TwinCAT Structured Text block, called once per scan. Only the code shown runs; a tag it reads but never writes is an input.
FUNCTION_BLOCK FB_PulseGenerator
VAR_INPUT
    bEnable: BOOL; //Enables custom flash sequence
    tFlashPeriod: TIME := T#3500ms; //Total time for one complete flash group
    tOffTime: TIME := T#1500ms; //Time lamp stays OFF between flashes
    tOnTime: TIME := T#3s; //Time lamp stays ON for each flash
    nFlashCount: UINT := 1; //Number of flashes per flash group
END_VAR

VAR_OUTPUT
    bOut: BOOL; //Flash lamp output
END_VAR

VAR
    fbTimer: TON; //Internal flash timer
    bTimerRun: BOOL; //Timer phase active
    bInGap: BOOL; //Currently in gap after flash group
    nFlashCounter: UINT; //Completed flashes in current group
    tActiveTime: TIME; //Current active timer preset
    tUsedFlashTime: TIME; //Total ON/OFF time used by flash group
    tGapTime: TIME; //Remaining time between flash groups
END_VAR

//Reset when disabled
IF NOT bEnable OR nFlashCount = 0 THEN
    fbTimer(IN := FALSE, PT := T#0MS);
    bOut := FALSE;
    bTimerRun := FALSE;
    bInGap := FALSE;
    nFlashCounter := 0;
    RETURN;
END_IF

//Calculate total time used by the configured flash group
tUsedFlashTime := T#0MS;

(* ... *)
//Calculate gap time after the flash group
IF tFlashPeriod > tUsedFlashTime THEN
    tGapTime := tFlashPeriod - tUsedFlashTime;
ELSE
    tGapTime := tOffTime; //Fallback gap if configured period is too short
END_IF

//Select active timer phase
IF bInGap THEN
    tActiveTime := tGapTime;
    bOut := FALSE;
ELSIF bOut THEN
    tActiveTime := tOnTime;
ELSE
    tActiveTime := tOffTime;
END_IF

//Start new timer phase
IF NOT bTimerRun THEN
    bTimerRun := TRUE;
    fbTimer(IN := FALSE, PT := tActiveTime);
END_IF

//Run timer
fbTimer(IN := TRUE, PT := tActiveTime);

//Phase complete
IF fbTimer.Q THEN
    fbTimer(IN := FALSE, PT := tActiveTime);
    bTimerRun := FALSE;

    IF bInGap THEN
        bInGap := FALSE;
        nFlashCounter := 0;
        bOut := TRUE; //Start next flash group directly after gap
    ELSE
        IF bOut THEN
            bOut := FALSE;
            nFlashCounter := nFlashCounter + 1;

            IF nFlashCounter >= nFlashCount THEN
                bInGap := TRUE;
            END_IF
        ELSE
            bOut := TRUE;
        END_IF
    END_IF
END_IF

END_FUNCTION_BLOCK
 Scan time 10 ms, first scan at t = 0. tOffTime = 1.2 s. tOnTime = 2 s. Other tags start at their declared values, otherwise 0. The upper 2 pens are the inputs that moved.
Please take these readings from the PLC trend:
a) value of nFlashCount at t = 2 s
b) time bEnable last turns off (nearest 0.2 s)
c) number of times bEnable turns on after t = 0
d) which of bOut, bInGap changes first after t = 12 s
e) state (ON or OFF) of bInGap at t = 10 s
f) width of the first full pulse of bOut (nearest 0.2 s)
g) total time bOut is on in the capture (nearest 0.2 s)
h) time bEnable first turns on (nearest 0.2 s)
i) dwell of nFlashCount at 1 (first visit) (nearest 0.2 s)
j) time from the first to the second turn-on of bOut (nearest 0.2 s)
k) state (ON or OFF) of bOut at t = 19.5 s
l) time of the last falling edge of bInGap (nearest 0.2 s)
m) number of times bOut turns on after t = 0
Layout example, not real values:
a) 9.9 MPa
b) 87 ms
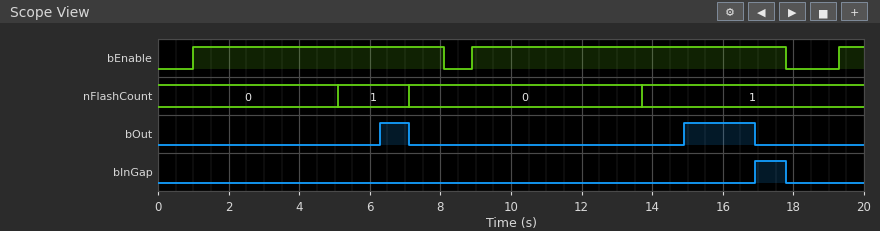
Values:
a) 0
b) 17.8 s
c) 3
d) bOut
e) OFF
f) 0.8 s
g) 2.8 s
h) 1.0 s
i) 2.0 s
j) 8.6 s
k) OFF
l) 17.8 s
m) 2
